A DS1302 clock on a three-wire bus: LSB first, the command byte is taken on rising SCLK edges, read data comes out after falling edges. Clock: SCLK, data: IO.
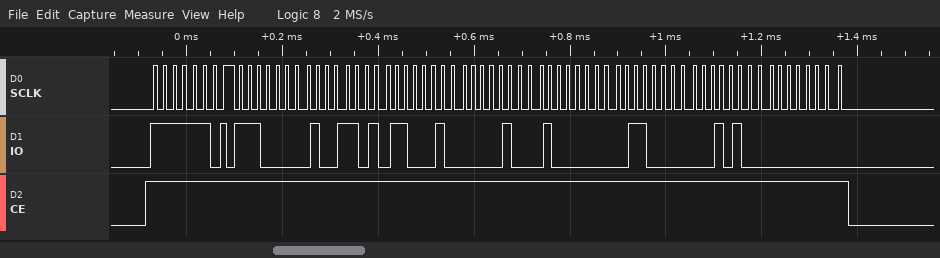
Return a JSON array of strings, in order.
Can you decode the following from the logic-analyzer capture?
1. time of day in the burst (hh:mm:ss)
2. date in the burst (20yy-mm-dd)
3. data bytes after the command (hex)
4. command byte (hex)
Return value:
["23:59:07", "2014-01-10", "07 59 23 10 01 06 14 00", "0xBF"]
